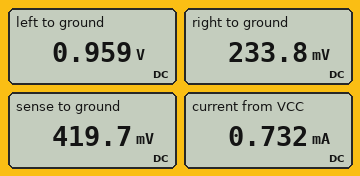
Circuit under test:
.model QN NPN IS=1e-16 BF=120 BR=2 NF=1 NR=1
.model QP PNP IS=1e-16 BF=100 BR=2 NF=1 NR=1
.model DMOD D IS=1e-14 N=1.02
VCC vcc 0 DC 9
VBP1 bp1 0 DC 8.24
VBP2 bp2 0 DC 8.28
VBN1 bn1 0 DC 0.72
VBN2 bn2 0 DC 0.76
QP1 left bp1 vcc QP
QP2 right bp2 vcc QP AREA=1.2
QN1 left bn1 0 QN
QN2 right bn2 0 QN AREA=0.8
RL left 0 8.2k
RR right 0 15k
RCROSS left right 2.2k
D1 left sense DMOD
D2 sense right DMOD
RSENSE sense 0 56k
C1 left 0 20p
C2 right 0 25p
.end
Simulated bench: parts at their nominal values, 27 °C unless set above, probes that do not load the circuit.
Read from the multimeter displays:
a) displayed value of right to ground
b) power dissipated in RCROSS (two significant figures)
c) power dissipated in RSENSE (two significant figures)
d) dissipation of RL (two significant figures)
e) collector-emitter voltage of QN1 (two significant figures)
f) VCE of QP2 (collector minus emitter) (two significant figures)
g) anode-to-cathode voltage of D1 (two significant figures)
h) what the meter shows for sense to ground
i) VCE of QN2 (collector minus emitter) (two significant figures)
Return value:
233.8 mV
240 µW
3.1 µW
110 µW
960 mV
-8.8 V
540 mV
419.7 mV
230 mV
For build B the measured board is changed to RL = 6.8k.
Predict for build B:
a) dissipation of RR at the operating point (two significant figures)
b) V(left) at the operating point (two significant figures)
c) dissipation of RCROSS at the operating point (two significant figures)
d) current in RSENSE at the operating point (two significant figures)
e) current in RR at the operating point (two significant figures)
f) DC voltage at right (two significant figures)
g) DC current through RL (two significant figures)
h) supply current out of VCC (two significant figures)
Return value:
1.5 µW
860 mV
230 µW
5.8 µA
9.9 µA
150 mV
130 µA
730 µA
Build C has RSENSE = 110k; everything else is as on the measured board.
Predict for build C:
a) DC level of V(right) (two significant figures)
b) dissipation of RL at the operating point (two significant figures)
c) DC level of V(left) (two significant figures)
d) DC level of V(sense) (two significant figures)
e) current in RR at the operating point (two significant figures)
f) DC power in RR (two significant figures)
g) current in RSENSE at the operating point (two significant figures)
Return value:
250 mV
120 µW
980 mV
450 mV
17 µA
4.2 µW
4.1 µA
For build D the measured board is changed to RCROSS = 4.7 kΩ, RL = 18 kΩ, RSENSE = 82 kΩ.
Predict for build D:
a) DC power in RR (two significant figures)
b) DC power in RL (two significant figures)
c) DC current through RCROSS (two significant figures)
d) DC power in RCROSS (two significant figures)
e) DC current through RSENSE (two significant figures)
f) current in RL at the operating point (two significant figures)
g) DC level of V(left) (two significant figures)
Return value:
16 µW
160 µW
260 µA
310 µW
13 µA
94 µA
1.7 V
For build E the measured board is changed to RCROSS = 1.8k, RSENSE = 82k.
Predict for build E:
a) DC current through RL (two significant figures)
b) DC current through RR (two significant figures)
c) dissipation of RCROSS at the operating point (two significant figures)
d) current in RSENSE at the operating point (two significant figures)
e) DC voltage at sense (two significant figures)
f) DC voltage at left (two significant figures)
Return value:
110 µA
22 µA
200 µW
4.9 µA
400 mV
930 mV
